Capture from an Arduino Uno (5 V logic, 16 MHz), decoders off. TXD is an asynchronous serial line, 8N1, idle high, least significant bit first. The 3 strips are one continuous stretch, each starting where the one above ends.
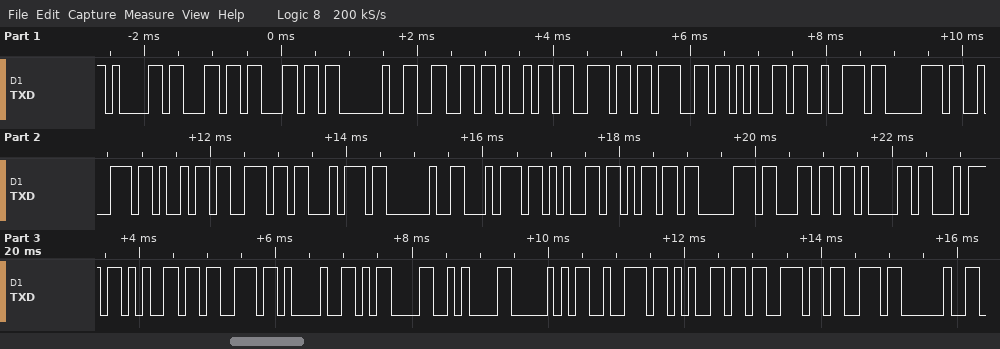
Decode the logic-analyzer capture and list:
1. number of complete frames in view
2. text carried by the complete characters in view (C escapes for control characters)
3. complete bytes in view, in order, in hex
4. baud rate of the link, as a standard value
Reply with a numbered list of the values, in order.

1. 34
2. "all fingerprint templates!\r\nPress "
3. 61 6C 6C 20 66 69 6E 67 65 72 70 72 69 6E 74 20 74 65 6D 70 6C 61 74 65 73 21 0D 0A 50 72 65 73 73 20
4. 9600 baud
